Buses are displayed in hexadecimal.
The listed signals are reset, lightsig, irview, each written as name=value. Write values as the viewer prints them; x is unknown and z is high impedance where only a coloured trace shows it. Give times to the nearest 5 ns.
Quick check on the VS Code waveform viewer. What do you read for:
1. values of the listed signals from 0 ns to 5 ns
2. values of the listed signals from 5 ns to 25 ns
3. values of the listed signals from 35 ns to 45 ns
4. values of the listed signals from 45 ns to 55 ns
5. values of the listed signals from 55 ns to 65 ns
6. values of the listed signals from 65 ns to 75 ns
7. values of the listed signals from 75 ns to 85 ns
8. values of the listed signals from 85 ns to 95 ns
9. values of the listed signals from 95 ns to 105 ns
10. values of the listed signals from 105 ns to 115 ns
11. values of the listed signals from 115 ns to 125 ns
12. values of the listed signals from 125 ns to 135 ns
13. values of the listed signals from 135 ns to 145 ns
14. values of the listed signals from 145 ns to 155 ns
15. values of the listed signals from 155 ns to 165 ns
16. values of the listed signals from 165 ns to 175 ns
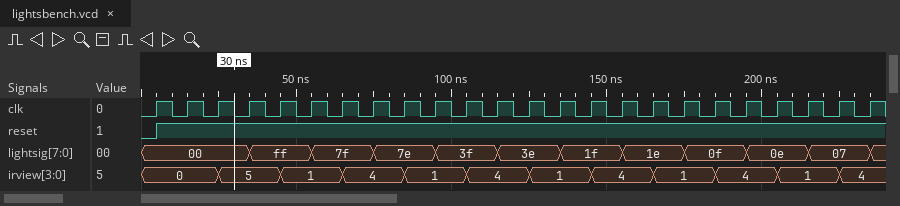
reset=0, lightsig=00, irview=0
reset=1, lightsig=00, irview=0
reset=1, lightsig=ff, irview=5
reset=1, lightsig=ff, irview=1
reset=1, lightsig=7f, irview=1
reset=1, lightsig=7f, irview=4
reset=1, lightsig=7e, irview=4
reset=1, lightsig=7e, irview=1
reset=1, lightsig=3f, irview=1
reset=1, lightsig=3f, irview=4
reset=1, lightsig=3e, irview=4
reset=1, lightsig=3e, irview=1
reset=1, lightsig=1f, irview=1
reset=1, lightsig=1f, irview=4
reset=1, lightsig=1e, irview=4
reset=1, lightsig=1e, irview=1
